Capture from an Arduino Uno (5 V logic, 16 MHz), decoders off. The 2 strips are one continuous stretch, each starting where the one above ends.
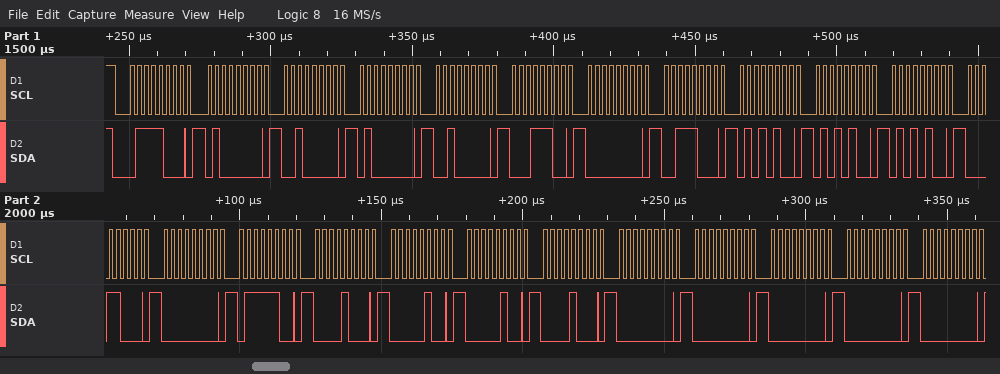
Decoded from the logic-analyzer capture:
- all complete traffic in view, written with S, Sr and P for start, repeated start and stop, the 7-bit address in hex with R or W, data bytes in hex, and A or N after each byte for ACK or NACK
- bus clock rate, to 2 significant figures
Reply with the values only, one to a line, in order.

S 3CW A 40 A 20 A 40 A 20 A 1C A 00 A 38 A 54 A 54 A 54 A 18 A 00 A 7C A 08 A 04 A 04 A 08 A 00 A 00 A 00 A 00 A 00 A
400 kHz
